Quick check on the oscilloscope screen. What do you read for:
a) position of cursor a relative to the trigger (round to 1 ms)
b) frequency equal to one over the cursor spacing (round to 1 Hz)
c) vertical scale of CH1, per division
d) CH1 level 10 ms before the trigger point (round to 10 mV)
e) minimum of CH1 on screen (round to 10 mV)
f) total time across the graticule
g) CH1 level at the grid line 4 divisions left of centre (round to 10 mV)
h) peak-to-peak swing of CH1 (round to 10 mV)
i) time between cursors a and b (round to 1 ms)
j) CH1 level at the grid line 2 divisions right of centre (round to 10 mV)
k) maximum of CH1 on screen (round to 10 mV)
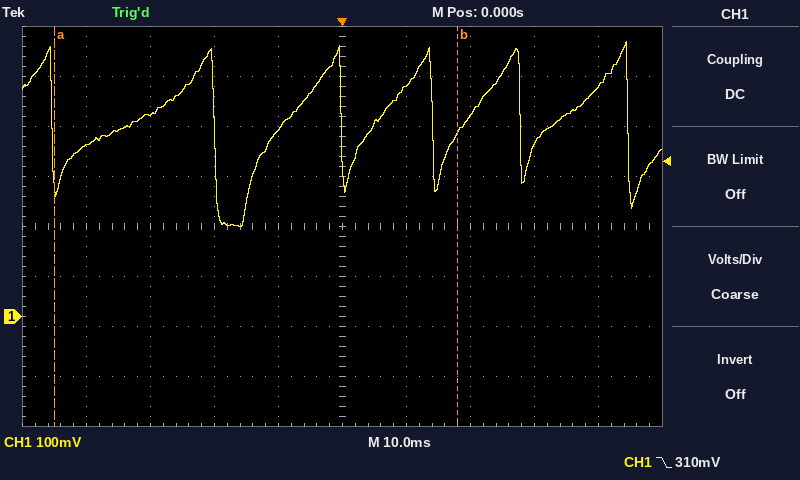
-45 ms
16 Hz
100 mV
370 mV
180 mV
100 ms
340 mV
370 mV
63 ms
400 mV
550 mV
